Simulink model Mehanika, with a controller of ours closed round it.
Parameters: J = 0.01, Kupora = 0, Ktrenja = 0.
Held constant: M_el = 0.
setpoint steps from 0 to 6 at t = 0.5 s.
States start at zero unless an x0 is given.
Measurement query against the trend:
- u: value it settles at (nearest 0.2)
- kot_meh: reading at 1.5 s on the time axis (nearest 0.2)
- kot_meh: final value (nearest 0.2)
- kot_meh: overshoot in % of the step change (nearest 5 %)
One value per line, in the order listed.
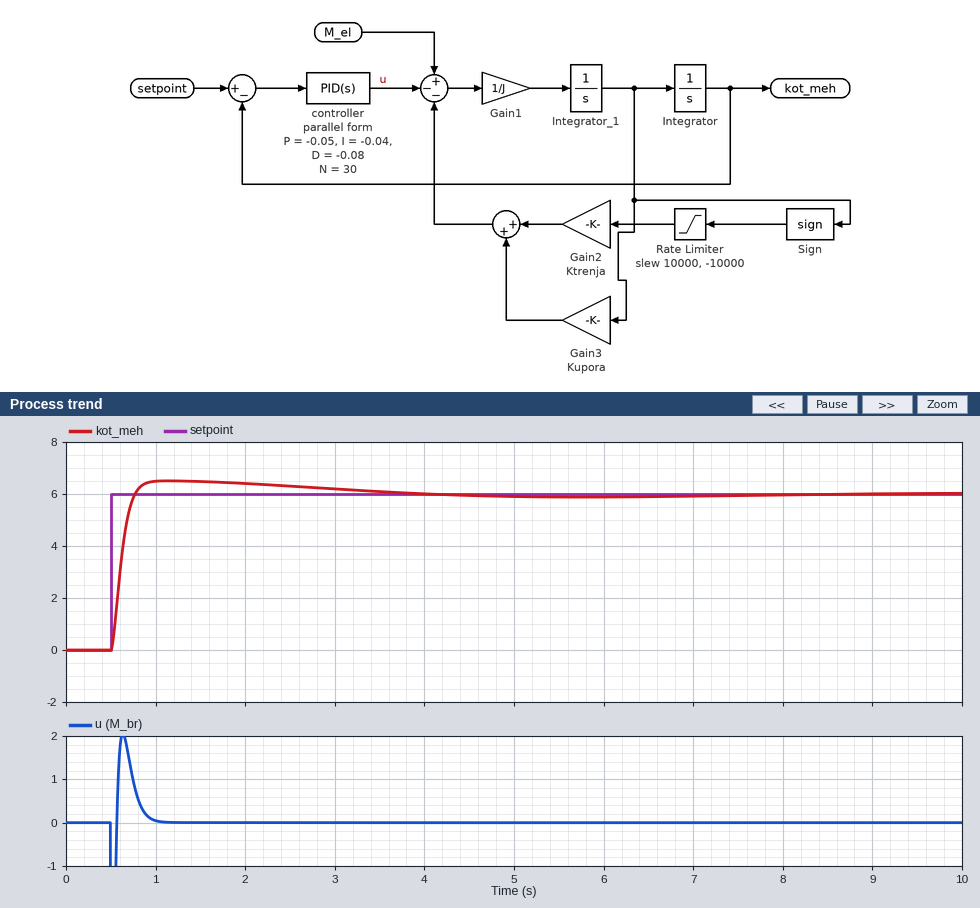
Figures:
0.0
6.4
6.0
10 %
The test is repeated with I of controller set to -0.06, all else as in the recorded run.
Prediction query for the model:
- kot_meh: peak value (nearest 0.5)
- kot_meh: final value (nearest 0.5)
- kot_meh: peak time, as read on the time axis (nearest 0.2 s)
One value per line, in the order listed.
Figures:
6.5
6.0
1.2 s
